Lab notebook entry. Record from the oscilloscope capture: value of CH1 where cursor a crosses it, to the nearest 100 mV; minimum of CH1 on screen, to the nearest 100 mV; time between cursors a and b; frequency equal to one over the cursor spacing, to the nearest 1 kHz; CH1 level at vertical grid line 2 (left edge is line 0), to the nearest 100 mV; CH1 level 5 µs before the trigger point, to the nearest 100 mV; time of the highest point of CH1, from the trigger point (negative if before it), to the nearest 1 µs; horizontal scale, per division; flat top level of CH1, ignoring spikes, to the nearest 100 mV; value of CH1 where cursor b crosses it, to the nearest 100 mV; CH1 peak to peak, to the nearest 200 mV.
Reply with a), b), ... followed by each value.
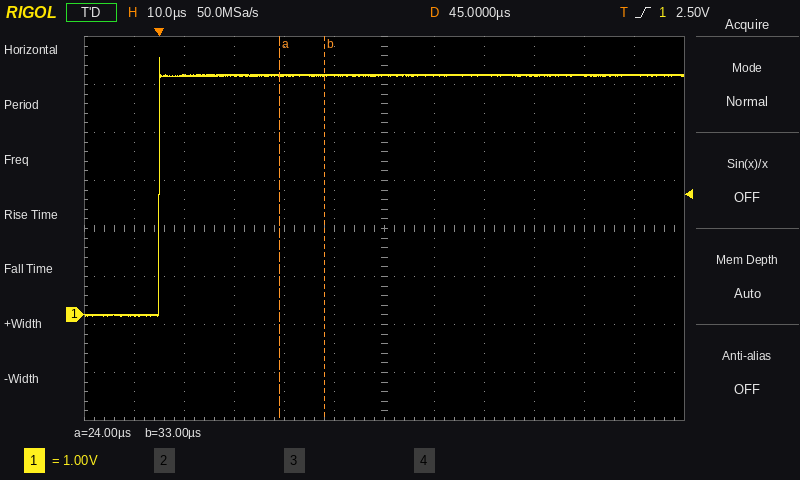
a) 5.0 V
b) 0.0 V
c) 9 µs
d) 111 kHz
e) 5.0 V
f) 0.0 V
g) 0 µs
h) 10 µs
i) 5.0 V
j) 5.0 V
k) 5.4 V
